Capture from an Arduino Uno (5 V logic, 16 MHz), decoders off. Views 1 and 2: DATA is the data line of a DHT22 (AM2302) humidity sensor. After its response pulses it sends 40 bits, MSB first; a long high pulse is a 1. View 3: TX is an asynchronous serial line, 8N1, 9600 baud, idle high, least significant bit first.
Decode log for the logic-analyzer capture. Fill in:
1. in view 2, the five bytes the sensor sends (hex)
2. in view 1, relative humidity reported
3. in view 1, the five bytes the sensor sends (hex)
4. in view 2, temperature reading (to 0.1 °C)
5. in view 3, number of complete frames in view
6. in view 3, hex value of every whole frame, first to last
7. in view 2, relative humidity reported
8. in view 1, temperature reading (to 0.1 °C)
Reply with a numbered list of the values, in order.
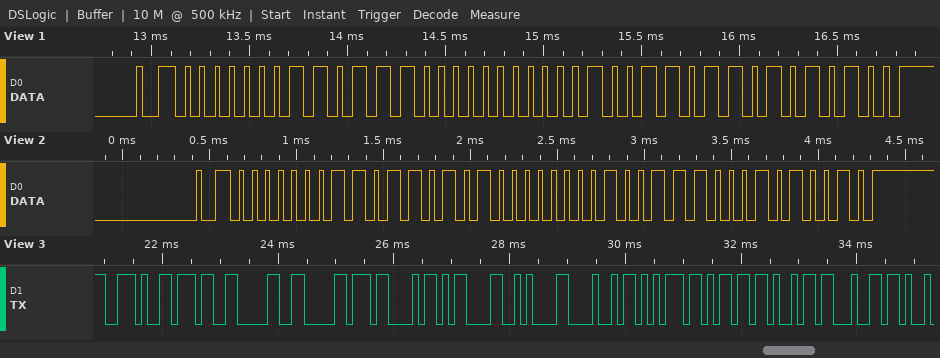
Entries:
1. 01 B5 00 9C 52
2. 44.0 %
3. 01 B8 00 9B 54
4. 15.6 °C
5. 12
6. 2E 37 30 B0 43 0D 0A 48 75 6D 69 64
7. 43.7 %
8. 15.5 °C
